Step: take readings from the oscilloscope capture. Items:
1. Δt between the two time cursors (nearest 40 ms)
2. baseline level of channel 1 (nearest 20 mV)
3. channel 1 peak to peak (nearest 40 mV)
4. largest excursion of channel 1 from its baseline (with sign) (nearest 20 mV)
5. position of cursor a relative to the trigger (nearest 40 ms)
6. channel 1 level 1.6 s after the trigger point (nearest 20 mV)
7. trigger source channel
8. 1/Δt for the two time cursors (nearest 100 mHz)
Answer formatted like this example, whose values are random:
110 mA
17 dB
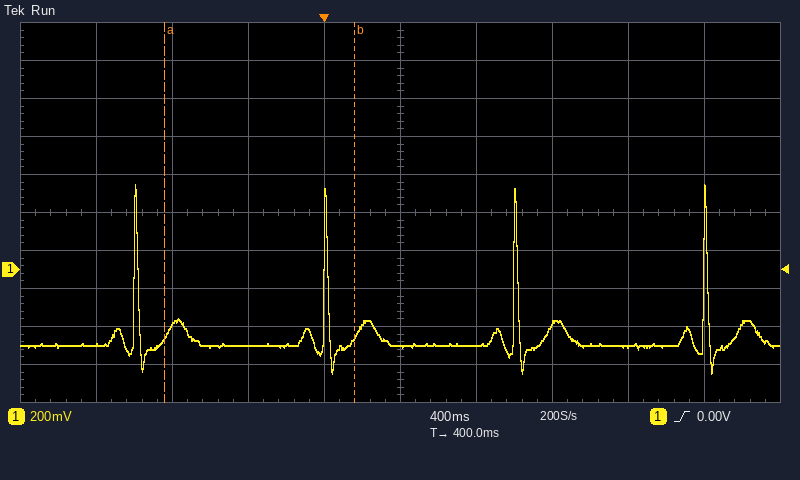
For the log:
1.00 s
-400 mV
1.00 V
+840 mV
-840 ms
-400 mV
channel 1
1.0 Hz
